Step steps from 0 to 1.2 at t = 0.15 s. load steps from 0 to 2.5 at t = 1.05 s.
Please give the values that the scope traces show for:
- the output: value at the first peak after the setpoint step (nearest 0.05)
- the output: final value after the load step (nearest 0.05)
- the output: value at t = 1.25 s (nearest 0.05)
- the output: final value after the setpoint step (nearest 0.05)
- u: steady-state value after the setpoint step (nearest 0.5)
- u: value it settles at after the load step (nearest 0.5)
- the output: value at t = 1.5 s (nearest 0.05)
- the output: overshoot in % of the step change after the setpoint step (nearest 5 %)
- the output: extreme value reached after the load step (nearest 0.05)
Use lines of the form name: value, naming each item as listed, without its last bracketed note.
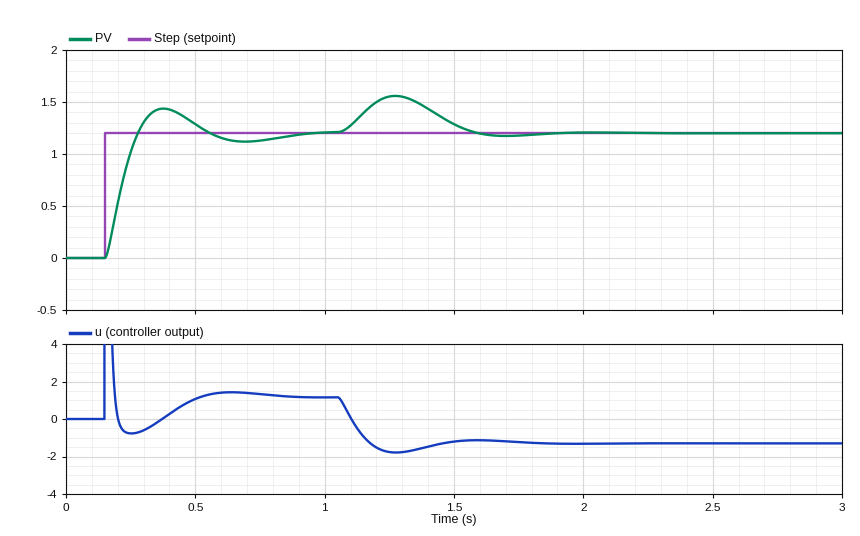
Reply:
the output: value at the first peak after the setpoint step: 1.45
the output: final value after the load step: 1.20
the output: value at t = 1.25 s: 1.55
the output: final value after the setpoint step: 1.20
u: steady-state value after the setpoint step: 1.0
u: value it settles at after the load step: -1.5
the output: value at t = 1.5 s: 1.30
the output: overshoot in % of the step change after the setpoint step: 20 %
the output: extreme value reached after the load step: 1.55
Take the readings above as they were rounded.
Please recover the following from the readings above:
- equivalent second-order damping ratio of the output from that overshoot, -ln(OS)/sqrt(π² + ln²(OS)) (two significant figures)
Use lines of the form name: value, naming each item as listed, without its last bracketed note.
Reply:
equivalent second-order damping ratio of the output from that overshoot, -ln(OS)/sqrt(π² + ln²(OS)): 0.46
